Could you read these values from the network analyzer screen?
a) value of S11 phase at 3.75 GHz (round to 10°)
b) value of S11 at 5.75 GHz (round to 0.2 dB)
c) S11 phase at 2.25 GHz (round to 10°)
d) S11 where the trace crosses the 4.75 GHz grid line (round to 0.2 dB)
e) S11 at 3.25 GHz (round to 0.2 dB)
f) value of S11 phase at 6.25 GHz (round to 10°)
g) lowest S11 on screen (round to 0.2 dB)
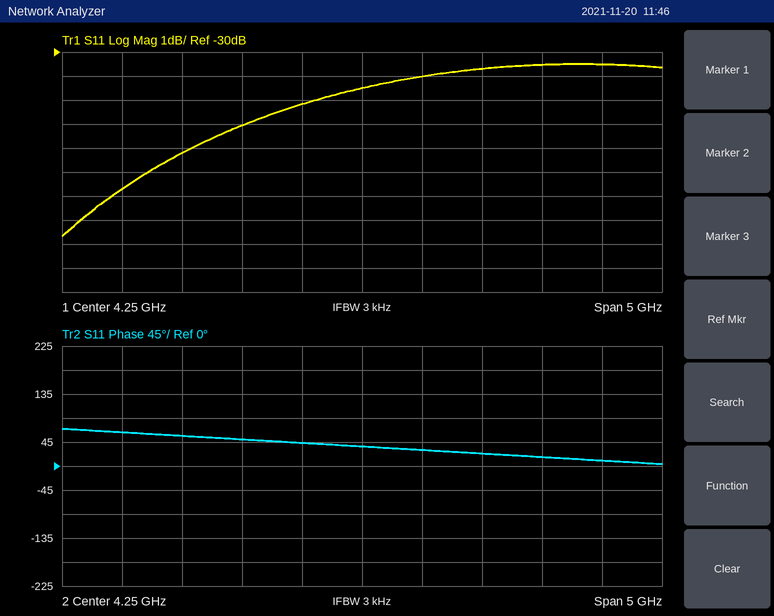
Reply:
40°
-30.6 dB
60°
-31.0 dB
-33.0 dB
10°
-37.6 dB
